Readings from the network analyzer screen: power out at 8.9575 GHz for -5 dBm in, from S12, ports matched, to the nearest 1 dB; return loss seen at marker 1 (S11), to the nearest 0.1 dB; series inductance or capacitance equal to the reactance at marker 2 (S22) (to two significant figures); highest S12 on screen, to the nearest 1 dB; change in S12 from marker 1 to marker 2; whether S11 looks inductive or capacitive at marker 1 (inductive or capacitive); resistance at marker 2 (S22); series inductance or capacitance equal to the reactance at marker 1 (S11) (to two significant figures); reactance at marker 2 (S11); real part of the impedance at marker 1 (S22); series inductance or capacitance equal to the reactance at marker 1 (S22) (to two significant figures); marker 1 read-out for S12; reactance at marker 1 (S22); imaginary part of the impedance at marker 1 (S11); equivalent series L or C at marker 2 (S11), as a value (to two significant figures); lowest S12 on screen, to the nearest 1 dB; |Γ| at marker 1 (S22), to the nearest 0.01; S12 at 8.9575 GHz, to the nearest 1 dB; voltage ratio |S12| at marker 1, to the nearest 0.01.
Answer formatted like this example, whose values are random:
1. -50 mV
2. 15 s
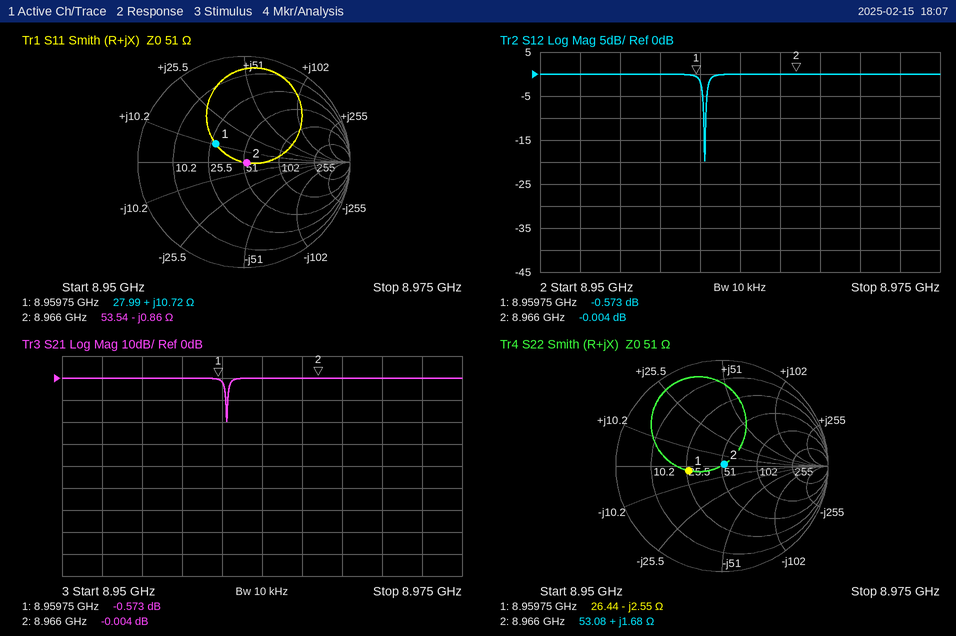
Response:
1. -5 dBm
2. 9.9 dB
3. 30 pH
4. 0 dB
5. 0.569 dB
6. inductive
7. 53.08 Ω
8. 190 pH
9. -0.86 Ω
10. 26.44 Ω
11. 7.0 pF
12. -0.573 dB
13. -2.55 Ω
14. +10.72 Ω
15. 21 pF
16. -20 dB
17. 0.32
18. 0 dB
19. 0.94
